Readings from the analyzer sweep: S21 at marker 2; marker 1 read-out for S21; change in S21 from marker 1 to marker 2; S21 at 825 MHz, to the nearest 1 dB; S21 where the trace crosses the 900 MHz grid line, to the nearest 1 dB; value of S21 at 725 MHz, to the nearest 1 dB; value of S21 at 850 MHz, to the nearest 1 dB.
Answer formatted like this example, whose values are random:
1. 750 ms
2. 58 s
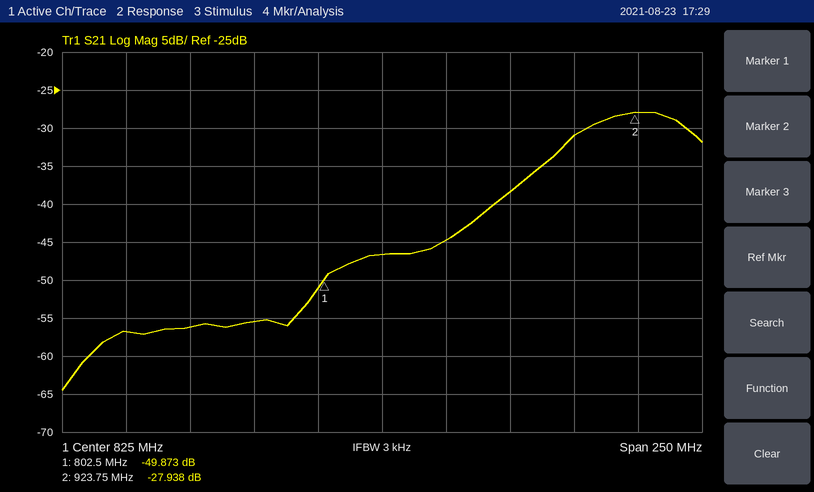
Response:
1. -27.938 dB
2. -49.873 dB
3. 21.935 dB
4. -47 dB
5. -31 dB
6. -57 dB
7. -45 dB
